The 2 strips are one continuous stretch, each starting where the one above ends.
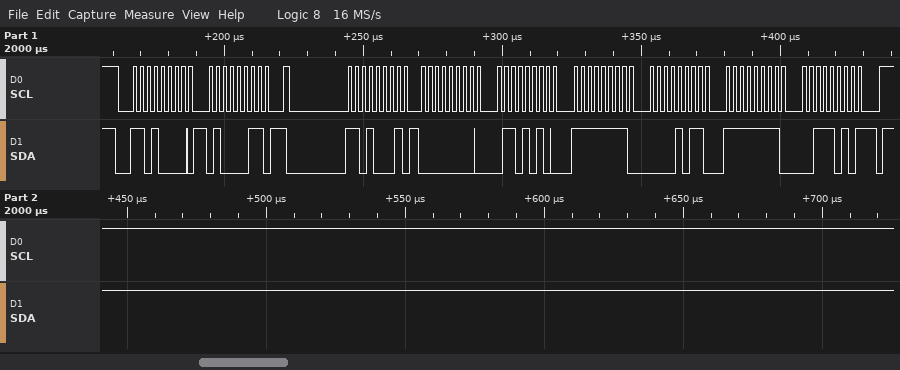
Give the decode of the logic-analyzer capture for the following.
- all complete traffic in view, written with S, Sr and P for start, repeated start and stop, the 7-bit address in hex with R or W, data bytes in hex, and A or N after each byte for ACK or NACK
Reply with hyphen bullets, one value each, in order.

- S 68W A 43 A Sr 68R A 00 A 6A A FF A 0B A FF A 3A N P
